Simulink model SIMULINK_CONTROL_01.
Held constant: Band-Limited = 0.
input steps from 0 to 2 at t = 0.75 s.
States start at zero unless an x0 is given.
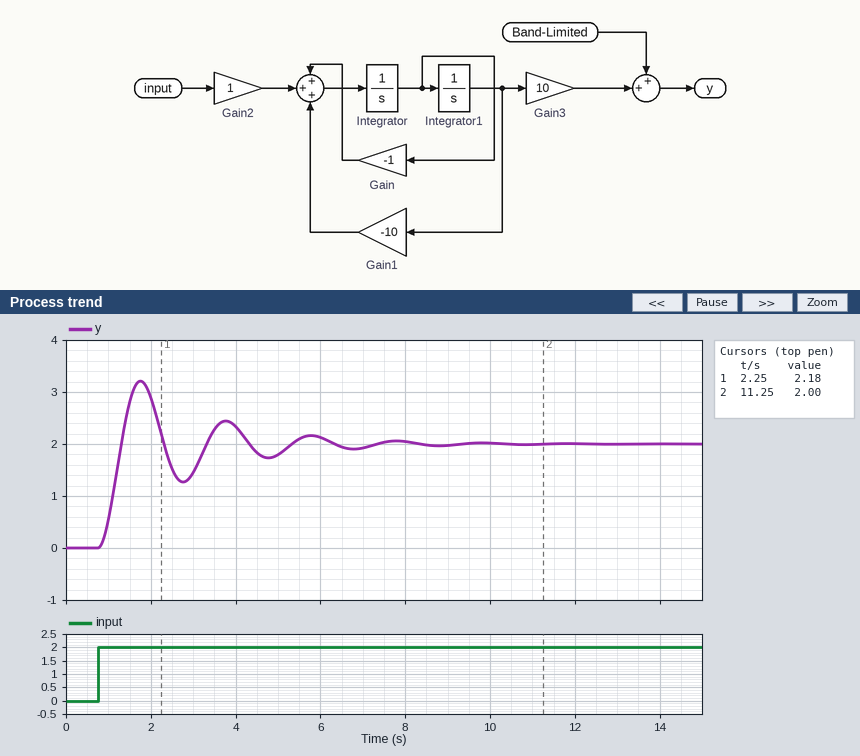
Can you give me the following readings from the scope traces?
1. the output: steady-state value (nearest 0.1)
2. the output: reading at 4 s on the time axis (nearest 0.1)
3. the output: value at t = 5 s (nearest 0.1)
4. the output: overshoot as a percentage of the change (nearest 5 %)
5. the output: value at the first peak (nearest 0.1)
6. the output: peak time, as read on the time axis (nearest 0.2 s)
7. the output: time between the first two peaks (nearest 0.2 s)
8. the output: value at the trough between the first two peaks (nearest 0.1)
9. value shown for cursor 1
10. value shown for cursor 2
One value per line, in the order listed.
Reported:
2.0
2.3
1.8
60 %
3.2
1.8 s
2.0 s
1.3
2.18
2.00
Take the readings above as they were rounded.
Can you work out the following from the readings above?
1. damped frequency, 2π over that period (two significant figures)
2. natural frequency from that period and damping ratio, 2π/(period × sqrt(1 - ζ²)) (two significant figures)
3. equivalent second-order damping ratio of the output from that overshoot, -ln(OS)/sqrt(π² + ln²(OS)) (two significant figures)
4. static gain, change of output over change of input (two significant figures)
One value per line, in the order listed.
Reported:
3.1 rad/s
3.2 rad/s
0.16
1.0
